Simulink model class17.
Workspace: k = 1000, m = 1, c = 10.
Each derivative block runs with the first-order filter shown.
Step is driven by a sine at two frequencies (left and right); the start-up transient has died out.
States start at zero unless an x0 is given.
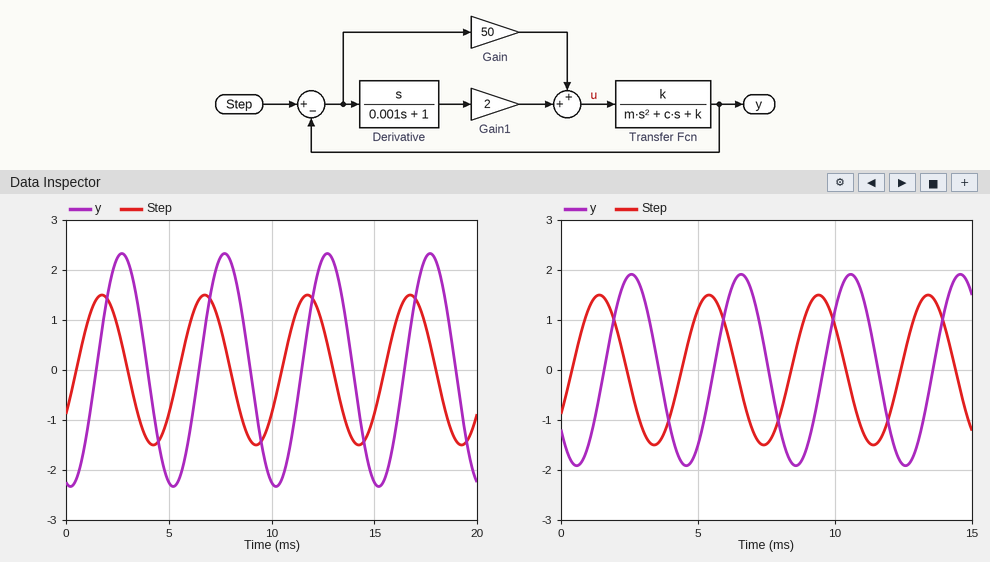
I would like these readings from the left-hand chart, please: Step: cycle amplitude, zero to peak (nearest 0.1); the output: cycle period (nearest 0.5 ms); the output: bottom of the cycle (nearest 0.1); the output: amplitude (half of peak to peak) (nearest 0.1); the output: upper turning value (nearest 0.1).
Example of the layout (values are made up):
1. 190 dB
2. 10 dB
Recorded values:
1. 1.5
2. 5.0 ms
3. -2.3
4. 2.3
5. 2.3
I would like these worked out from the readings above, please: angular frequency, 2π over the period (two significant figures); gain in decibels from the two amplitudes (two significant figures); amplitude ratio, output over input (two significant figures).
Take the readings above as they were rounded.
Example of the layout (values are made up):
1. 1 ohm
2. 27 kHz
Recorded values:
1. 1.3 rad/ms
2. 3.7 dB
3. 1.5
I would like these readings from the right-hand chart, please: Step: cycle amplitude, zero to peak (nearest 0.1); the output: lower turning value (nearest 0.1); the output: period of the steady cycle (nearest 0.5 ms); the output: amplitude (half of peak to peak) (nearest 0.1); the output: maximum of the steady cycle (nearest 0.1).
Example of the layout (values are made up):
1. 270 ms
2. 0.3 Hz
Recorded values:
1. 1.5
2. -1.9
3. 4.0 ms
4. 1.9
5. 1.9
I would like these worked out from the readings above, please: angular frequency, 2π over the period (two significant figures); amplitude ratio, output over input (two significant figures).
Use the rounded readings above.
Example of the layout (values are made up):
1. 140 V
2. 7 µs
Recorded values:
1. 1.6 rad/ms
2. 1.3
